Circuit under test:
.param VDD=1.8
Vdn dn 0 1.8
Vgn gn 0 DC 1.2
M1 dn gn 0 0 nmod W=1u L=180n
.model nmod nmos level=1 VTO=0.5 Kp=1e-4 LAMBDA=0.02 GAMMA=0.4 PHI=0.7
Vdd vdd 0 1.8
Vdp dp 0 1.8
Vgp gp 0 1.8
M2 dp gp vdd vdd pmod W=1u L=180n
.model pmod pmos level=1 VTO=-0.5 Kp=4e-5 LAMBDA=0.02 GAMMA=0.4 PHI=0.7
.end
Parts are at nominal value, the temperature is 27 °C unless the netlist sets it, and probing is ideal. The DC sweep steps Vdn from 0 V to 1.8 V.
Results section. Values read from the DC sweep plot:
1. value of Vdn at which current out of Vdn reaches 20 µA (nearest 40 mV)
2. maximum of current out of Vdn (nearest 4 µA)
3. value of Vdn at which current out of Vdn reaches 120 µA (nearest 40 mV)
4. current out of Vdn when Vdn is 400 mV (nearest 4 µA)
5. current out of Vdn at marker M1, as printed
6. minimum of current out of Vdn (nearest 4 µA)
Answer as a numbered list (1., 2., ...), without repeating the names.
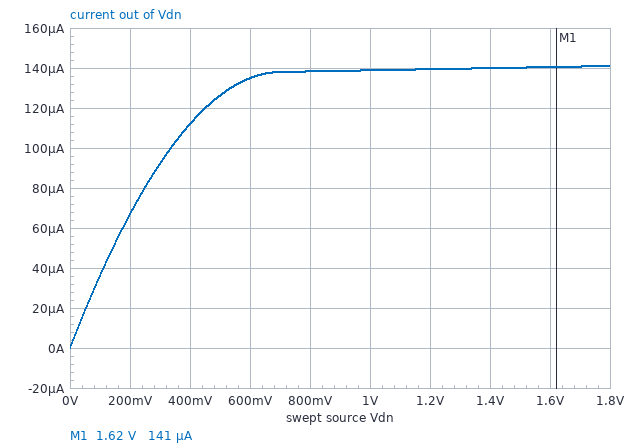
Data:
1. 40 mV
2. 140 µA
3. 440 mV
4. 112 µA
5. 141 µA
6. 0 A
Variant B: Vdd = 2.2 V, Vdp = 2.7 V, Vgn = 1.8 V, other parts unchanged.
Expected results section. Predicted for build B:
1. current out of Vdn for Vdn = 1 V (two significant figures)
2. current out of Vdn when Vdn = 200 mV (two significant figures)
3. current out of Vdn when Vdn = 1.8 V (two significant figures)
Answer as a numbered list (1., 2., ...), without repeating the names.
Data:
1. 450 µA
2. 130 µA
3. 490 µA
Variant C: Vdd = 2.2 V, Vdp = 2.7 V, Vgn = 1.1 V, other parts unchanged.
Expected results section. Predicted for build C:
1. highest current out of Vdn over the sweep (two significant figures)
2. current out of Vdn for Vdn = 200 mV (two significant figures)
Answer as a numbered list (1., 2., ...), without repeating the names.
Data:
1. 100 µA
2. 56 µA
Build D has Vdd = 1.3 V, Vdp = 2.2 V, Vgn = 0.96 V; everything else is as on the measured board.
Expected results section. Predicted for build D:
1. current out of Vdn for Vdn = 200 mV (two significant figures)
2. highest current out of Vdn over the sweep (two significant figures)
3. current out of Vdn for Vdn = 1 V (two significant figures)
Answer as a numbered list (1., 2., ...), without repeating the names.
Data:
1. 40 µA
2. 61 µA
3. 60 µA
